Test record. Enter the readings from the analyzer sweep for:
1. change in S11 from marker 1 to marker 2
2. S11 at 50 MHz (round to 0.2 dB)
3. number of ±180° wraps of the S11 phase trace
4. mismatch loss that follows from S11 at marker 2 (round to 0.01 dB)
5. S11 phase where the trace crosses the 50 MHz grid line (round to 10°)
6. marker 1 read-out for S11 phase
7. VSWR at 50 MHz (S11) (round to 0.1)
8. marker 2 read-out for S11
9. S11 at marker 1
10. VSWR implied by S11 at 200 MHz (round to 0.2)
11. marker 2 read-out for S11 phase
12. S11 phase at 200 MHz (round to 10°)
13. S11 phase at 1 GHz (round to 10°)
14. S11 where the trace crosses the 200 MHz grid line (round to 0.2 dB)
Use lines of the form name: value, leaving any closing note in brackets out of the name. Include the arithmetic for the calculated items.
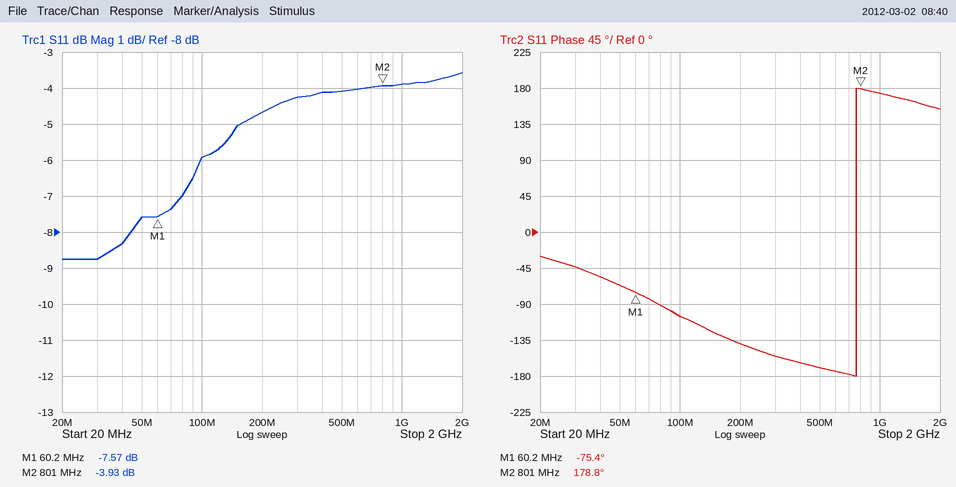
change in S11 from marker 1 to marker 2: -3.93 − (-7.57) = 3.64 dB
S11 at 50 MHz: -7.6 dB
number of ±180° wraps of the S11 phase trace: 1
mismatch loss that follows from S11 at marker 2: −10 log10(1 − 10^(-3.93/10)) ≈ 2.25 dB
S11 phase where the trace crosses the 50 MHz grid line: -70°
marker 1 read-out for S11 phase: -75.4°
VSWR at 50 MHz (S11): |Γ| = 10^(-7.6/20) = 0.4169; VSWR = (1 + 0.4169)/(1 − 0.4169) ≈ 2.4
marker 2 read-out for S11: -3.93 dB
S11 at marker 1: -7.57 dB
VSWR implied by S11 at 200 MHz: |Γ| = 10^(-4.6/20) = 0.5888; VSWR = (1 + 0.5888)/(1 − 0.5888) ≈ 3.86, so 3.8 to the nearest 0.2
marker 2 read-out for S11 phase: 178.8°
S11 phase at 200 MHz: -140°
S11 phase at 1 GHz: 170°
S11 where the trace crosses the 200 MHz grid line: -4.6 dB
